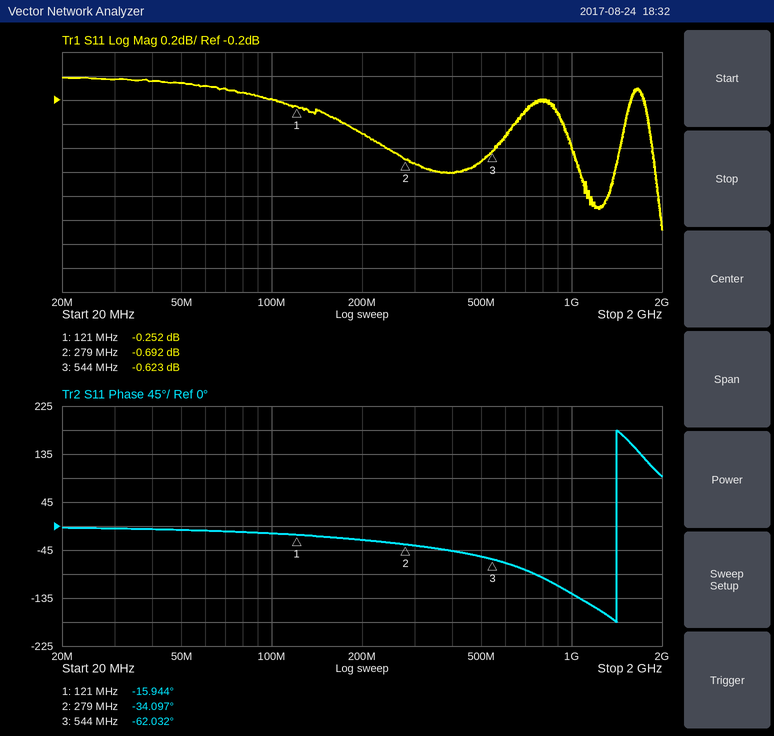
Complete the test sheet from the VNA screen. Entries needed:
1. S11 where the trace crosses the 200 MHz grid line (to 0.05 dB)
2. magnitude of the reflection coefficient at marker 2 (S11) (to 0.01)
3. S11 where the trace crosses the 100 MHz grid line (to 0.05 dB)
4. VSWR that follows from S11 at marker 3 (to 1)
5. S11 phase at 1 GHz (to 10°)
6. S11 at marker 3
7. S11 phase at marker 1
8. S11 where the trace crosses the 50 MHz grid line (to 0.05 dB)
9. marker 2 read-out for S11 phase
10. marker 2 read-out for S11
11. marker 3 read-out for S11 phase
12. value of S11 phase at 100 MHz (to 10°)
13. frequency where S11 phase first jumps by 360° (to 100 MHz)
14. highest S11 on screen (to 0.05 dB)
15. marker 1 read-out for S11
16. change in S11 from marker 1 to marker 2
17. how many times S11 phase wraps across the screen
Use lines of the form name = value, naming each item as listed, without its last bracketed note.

S11 where the trace crosses the 200 MHz grid line = -0.50 dB
magnitude of the reflection coefficient at marker 2 (S11) = 0.92
S11 where the trace crosses the 100 MHz grid line = -0.20 dB
VSWR that follows from S11 at marker 3 = 28
S11 phase at 1 GHz = -130°
S11 at marker 3 = -0.623 dB
S11 phase at marker 1 = -15.944°
S11 where the trace crosses the 50 MHz grid line = -0.05 dB
marker 2 read-out for S11 phase = -34.097°
marker 2 read-out for S11 = -0.692 dB
marker 3 read-out for S11 phase = -62.032°
value of S11 phase at 100 MHz = -10°
frequency where S11 phase first jumps by 360° = 1.4 GHz
highest S11 on screen = 0.00 dB
marker 1 read-out for S11 = -0.252 dB
change in S11 from marker 1 to marker 2 = -0.440 dB
how many times S11 phase wraps across the screen = 1
